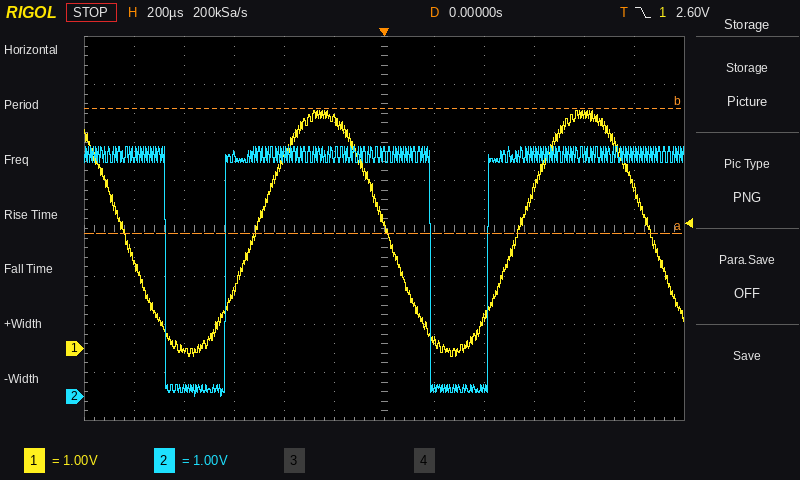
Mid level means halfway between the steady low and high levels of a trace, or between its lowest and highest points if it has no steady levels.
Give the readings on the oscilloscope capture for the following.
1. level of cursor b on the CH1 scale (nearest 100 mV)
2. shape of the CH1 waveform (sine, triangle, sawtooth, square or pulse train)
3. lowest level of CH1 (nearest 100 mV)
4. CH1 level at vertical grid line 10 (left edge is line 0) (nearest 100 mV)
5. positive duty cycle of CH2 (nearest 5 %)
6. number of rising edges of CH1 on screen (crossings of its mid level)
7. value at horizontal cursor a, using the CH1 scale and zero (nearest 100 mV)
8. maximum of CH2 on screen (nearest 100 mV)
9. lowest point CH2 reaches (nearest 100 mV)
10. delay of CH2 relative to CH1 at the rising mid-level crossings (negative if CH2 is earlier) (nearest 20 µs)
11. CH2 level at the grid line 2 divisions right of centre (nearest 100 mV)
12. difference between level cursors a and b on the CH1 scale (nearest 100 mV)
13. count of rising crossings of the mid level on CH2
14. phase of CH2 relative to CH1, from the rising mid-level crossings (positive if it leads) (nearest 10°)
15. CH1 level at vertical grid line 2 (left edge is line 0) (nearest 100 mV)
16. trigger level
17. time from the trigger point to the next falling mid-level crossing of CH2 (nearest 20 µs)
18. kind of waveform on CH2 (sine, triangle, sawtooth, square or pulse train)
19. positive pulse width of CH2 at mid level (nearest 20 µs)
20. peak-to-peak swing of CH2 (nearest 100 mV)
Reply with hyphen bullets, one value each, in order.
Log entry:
- 5.0 V
- sine
- -200 mV
- 4.9 V
- 80 %
- 2
- 2.4 V
- 5.2 V
- 0.0 V
- -120 µs
- 200 mV
- 2.6 V
- 2
- +40°
- 0.0 V
- 2.60 V
- 180 µs
- pulse train
- 820 µs
- 5.2 V
